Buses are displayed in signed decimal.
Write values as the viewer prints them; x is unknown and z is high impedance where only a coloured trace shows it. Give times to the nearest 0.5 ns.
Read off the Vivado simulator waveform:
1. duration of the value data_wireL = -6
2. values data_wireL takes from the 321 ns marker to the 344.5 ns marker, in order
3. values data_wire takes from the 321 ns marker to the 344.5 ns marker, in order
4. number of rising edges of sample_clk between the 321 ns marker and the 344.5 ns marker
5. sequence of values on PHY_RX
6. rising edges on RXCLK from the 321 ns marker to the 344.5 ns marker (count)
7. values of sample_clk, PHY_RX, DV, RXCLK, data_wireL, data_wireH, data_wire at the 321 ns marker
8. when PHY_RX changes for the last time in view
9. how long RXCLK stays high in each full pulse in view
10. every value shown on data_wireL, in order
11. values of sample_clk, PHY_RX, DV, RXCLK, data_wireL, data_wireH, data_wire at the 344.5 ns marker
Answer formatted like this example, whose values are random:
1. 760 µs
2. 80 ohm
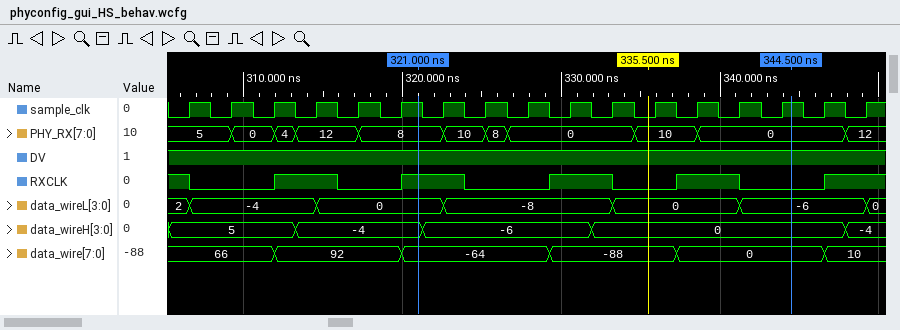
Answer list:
1. 8 ns
2. 0, -8, 0, -6
3. -64, -88, 0
4. 9
5. 5, 0, 4, 12, 8, 10, 8, 0, 10, 0, 12
6. 2
7. sample_clk=1, PHY_RX=8, DV=1, RXCLK=1, data_wireL=0, data_wireH=-4, data_wire=-64
8. 348 ns
9. 4 ns, 4 ns, 4 ns, 4 ns
10. 2, -4, 0, -8, 0, -6, 0
11. sample_clk=1, PHY_RX=0, DV=1, RXCLK=0, data_wireL=-6, data_wireH=0, data_wire=0
